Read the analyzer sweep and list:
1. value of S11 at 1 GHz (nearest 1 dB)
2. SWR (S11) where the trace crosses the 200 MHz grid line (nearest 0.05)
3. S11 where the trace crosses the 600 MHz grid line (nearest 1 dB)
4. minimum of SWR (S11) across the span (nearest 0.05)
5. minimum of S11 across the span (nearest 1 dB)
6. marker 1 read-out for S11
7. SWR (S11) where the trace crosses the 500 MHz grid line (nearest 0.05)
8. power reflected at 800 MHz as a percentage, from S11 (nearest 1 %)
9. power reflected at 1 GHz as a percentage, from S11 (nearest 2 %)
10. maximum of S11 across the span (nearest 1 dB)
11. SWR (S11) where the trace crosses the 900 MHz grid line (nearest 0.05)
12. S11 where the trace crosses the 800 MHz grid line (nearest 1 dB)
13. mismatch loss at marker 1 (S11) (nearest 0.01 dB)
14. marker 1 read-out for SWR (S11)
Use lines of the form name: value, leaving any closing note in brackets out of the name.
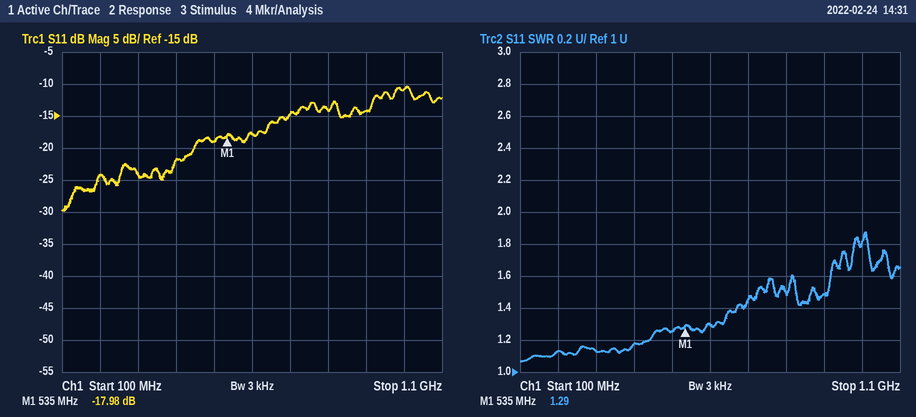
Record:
value of S11 at 1 GHz: -11 dB
SWR (S11) where the trace crosses the 200 MHz grid line: 1.15
S11 where the trace crosses the 600 MHz grid line: -18 dB
minimum of SWR (S11) across the span: 1.05
minimum of S11 across the span: -30 dB
marker 1 read-out for S11: -17.98 dB
SWR (S11) where the trace crosses the 500 MHz grid line: 1.25
power reflected at 800 MHz as a percentage, from S11: 4 %
power reflected at 1 GHz as a percentage, from S11: 8 %
maximum of S11 across the span: -10 dB
SWR (S11) where the trace crosses the 900 MHz grid line: 1.50
S11 where the trace crosses the 800 MHz grid line: -14 dB
mismatch loss at marker 1 (S11): 0.07 dB
marker 1 read-out for SWR: 1.29
